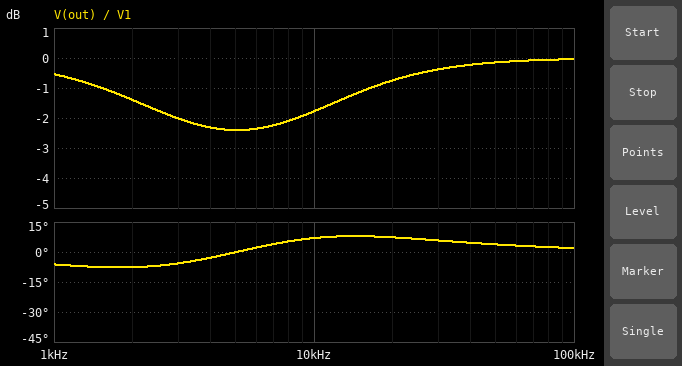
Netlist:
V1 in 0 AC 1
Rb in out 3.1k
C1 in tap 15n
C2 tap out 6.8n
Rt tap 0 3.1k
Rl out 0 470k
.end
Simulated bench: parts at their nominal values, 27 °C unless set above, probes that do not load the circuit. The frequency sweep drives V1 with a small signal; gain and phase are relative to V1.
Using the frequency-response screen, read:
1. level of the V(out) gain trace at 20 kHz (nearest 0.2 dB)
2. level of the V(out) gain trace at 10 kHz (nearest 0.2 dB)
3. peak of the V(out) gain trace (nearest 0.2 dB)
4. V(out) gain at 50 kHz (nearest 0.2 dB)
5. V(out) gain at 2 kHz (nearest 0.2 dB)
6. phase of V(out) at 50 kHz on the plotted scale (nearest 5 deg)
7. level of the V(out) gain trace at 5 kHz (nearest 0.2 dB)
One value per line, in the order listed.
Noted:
-0.8 dB
-1.8 dB
0 dB
-0.2 dB
-1.4 dB
5 deg
-2.4 dB
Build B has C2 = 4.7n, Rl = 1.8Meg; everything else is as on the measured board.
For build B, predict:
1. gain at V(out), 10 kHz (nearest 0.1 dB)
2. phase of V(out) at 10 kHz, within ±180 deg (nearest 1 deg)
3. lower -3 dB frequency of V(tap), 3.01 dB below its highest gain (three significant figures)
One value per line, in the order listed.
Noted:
-1.6 dB
4 deg
2.80 kHz
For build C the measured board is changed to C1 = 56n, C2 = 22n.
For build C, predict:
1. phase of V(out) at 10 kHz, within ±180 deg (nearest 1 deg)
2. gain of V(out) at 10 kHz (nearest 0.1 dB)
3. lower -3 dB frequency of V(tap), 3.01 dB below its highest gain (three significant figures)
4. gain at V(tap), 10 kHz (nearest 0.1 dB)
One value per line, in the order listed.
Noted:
5 deg
-0.3 dB
733 Hz
-0.1 dB
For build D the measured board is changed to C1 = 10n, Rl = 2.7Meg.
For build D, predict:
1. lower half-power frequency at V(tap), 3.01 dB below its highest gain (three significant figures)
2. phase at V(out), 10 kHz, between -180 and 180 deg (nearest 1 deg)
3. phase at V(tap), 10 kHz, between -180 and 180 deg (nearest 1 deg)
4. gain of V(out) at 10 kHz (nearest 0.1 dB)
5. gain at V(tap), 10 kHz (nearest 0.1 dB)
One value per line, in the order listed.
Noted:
3.93 kHz
7 deg
19 deg
-2.5 dB
-1.3 dB
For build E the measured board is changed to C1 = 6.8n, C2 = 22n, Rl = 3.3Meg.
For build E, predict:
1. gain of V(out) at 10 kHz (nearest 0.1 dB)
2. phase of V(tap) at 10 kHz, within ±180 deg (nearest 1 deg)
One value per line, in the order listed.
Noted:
-3.5 dB
20 deg
